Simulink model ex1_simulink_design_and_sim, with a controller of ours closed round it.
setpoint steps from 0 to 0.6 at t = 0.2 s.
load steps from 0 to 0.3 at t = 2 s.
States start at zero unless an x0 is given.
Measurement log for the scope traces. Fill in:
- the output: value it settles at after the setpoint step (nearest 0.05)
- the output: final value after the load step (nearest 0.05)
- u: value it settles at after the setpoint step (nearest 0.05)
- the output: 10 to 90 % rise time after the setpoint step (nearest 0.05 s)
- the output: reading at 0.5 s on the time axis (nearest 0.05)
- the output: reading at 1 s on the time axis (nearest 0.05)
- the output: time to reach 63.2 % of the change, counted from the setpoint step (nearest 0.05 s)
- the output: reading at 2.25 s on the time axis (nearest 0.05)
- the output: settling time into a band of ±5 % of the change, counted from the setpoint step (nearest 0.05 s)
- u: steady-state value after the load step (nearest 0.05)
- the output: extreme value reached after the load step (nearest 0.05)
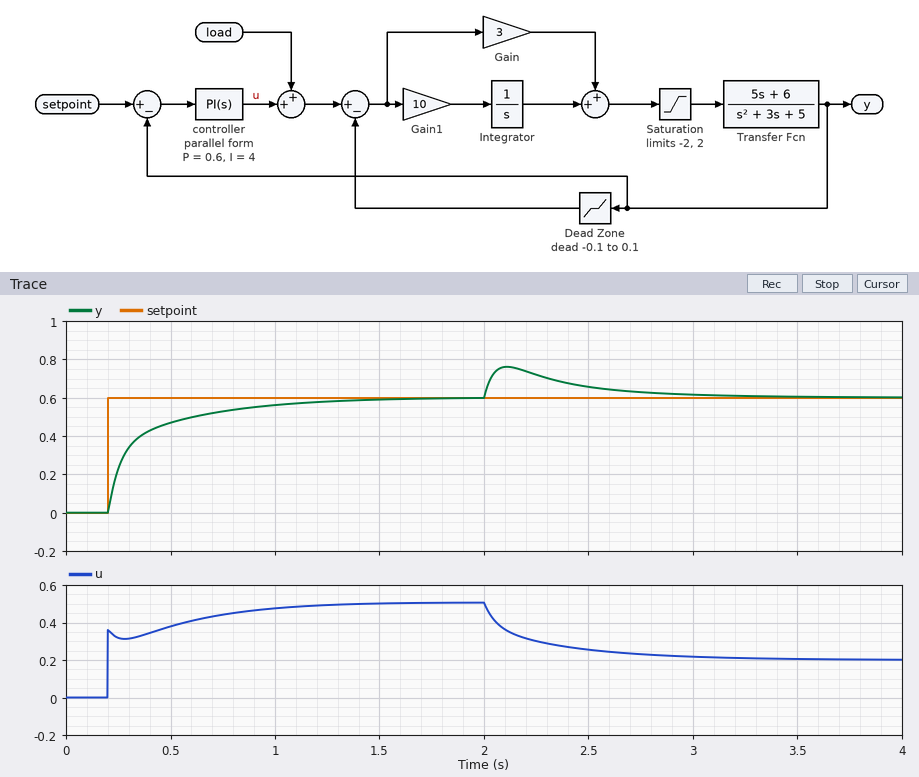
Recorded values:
0.60
0.60
0.50
0.60 s
0.45
0.55
0.15 s
0.70
0.90 s
0.20
0.75
